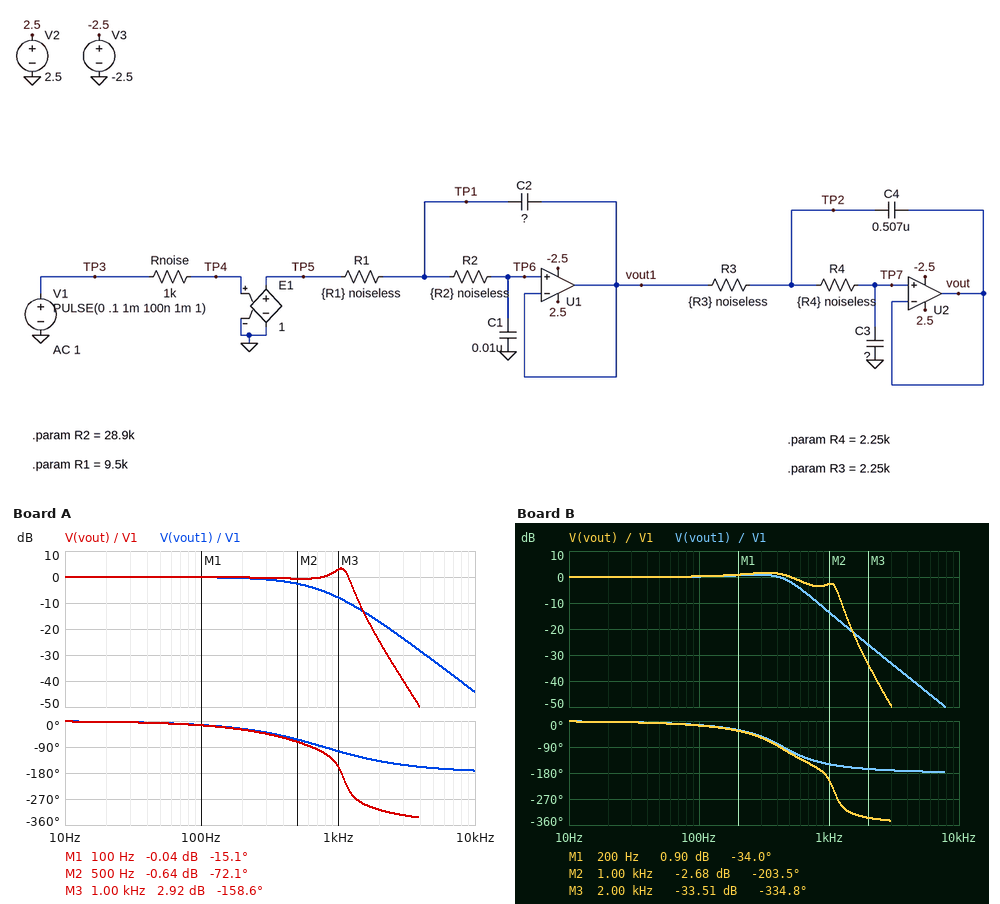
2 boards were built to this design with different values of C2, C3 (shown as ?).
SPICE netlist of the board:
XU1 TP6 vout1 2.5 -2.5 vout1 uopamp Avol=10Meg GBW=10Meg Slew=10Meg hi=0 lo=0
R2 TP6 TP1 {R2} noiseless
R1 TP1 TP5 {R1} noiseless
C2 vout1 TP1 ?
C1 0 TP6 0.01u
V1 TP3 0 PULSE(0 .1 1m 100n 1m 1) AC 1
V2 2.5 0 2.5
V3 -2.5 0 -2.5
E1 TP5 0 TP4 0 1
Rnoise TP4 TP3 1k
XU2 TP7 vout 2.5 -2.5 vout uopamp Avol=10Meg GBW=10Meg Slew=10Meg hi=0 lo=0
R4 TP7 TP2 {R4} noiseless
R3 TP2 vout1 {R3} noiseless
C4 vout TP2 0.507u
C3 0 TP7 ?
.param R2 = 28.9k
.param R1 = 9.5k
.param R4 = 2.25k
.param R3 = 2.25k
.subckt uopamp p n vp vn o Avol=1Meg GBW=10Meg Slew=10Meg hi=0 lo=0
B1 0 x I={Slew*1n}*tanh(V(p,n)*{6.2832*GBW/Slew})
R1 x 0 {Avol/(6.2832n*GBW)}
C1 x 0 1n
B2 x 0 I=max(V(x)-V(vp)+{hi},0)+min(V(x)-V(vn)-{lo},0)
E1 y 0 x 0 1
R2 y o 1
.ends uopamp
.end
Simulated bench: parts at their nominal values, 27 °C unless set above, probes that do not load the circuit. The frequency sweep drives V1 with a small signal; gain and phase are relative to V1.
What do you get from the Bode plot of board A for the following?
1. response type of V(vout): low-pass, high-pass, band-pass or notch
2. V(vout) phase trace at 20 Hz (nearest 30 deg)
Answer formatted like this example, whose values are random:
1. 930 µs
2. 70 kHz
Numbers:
1. low-pass
2. 0 deg
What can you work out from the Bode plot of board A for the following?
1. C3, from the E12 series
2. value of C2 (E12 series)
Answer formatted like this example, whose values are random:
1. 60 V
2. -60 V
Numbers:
1. 8.2 nF
2. 15 nF
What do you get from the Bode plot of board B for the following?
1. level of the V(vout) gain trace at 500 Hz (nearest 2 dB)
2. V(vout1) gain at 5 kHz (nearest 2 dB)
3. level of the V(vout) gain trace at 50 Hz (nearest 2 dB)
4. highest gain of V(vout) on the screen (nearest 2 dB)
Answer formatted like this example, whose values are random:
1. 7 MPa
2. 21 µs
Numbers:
1. 0 dB
2. -42 dB
3. 0 dB
4. 2 dB
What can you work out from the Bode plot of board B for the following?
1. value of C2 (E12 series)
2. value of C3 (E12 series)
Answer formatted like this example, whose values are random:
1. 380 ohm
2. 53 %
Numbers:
1. 47 nF
2. 8.2 nF
